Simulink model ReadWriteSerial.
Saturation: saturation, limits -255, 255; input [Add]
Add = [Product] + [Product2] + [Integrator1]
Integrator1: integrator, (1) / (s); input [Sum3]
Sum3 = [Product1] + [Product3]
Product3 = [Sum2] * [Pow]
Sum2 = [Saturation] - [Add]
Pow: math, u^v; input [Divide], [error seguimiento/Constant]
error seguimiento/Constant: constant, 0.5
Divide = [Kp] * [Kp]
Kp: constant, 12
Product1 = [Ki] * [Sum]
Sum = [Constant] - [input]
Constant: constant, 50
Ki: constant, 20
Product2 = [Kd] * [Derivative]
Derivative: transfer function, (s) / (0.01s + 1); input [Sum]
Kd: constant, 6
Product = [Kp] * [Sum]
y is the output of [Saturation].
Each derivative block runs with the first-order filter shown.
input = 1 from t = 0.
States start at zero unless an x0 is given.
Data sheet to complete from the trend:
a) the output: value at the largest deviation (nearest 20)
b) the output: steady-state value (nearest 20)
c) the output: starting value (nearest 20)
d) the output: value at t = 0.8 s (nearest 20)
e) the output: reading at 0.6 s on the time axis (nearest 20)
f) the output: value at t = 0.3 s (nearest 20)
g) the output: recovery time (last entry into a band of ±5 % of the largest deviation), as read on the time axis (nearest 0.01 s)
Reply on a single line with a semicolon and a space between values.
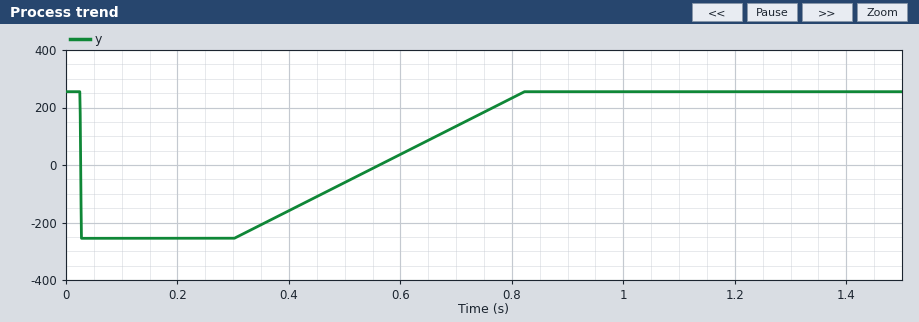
-260; 260; 260; 240; 40; -260; 0.80 s
